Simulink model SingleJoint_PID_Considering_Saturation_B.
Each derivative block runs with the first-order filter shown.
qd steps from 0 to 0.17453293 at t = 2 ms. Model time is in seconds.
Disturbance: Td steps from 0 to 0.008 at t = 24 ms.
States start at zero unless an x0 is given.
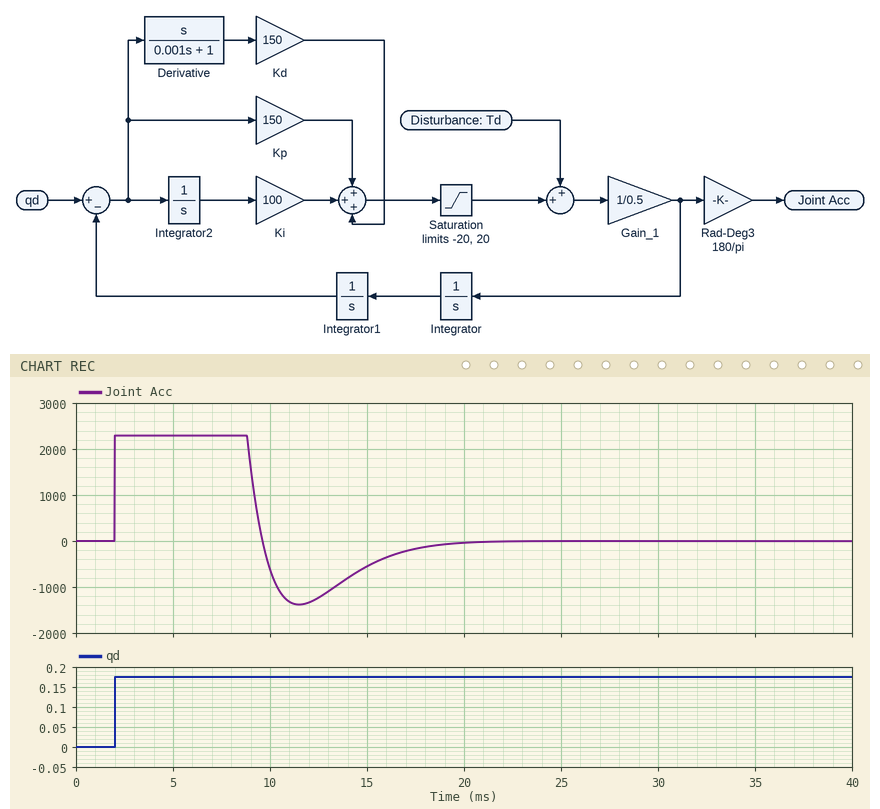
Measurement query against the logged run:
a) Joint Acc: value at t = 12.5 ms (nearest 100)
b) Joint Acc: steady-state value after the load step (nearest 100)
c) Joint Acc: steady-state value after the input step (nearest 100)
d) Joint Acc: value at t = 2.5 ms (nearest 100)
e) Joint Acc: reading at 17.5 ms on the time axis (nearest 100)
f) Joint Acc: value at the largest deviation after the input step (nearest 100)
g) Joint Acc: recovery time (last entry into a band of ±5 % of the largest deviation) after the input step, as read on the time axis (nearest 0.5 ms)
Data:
-1200
0
0
2300
-200
2300
18.0 ms
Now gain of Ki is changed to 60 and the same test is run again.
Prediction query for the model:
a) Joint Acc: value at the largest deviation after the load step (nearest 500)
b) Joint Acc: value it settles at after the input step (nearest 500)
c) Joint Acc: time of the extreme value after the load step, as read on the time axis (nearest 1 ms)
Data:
0
0
25 ms
